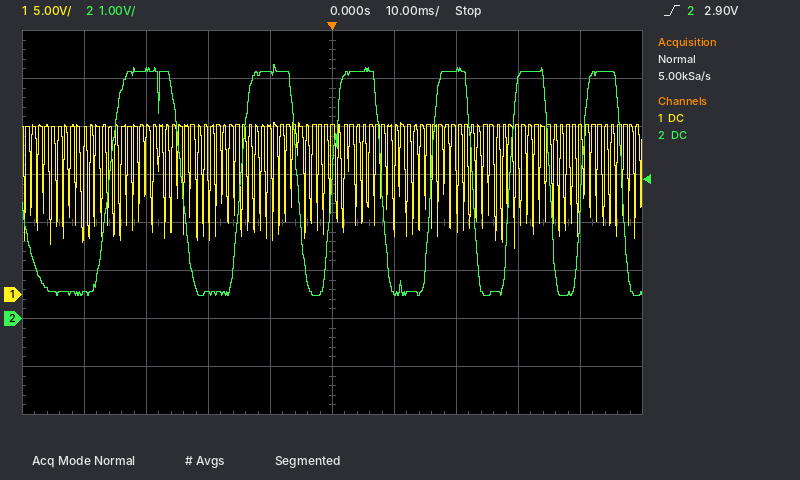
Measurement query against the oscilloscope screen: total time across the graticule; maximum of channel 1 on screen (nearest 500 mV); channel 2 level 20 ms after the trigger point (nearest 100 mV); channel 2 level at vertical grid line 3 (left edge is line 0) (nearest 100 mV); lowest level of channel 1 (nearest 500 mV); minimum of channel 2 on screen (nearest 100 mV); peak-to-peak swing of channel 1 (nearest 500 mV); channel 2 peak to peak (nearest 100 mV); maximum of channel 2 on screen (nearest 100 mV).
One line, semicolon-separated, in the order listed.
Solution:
100 ms; 18.0 V; 5.2 V; 500 mV; 5.0 V; 500 mV; 13.0 V; 4.8 V; 5.3 V
